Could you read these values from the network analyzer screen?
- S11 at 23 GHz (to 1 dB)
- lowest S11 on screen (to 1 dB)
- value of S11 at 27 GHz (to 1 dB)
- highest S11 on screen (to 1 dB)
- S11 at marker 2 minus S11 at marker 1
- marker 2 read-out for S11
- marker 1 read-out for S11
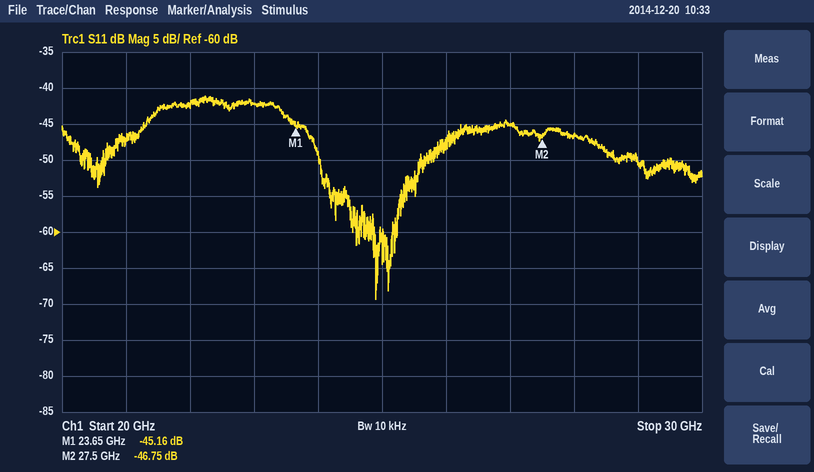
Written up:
-42 dB
-69 dB
-45 dB
-41 dB
-1.59 dB
-46.75 dB
-45.16 dB
